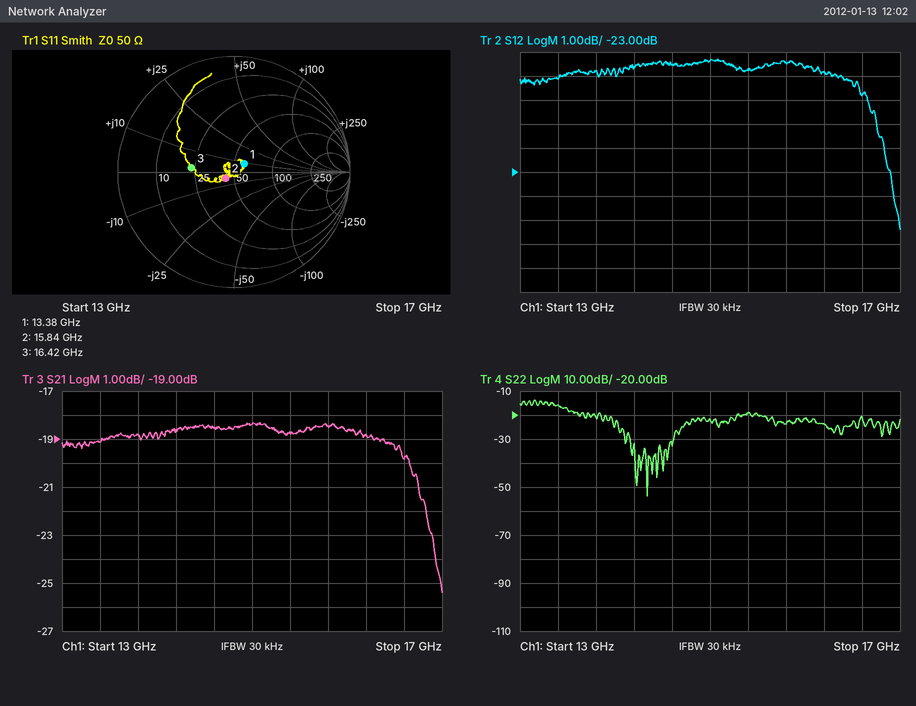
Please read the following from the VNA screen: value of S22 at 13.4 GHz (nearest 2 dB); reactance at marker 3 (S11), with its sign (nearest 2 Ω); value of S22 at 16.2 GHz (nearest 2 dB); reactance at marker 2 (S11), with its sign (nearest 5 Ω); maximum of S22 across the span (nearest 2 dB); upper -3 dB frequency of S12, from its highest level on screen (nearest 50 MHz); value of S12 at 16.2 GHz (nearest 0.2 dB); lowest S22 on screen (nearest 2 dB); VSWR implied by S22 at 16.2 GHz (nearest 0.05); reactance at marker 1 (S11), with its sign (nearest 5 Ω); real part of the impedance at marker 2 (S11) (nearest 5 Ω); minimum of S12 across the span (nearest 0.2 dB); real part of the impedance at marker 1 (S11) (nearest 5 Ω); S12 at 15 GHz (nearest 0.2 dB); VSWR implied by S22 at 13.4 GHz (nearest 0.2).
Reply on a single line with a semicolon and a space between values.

-16 dB; +2 Ω; -24 dB; -5 Ω; -14 dB; 16.75 GHz; -18.8 dB; -54 dB; 1.15; +10 Ω; 45 Ω; -25.4 dB; 60 Ω; -18.4 dB; 1.4
